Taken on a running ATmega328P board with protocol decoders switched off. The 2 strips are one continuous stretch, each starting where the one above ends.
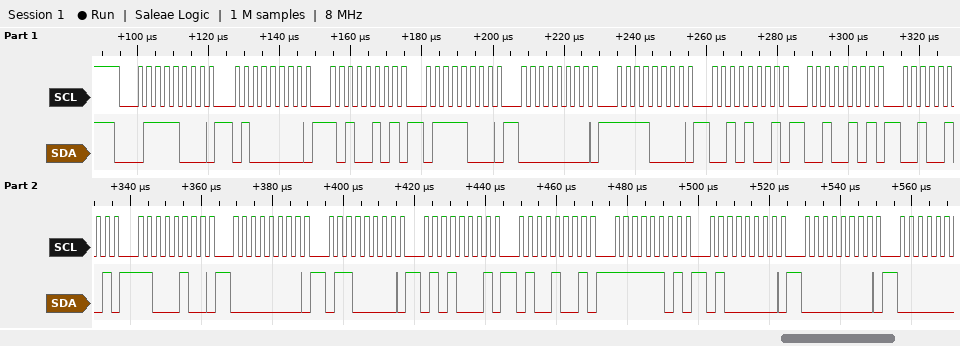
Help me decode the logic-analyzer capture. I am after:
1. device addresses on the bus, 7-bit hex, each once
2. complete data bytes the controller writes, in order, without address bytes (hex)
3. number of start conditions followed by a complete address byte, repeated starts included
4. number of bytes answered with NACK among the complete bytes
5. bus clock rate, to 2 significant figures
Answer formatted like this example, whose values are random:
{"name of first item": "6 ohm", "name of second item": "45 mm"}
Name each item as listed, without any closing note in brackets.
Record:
{"device addresses on the bus, 7-bit hex, each once": "0x3C", "complete data bytes the controller writes, in order, without address bytes": "40 A5 78 00 F0 29 25 25 C4 00 60 51 49 FD 40 00", "number of start conditions followed by a complete address byte, repeated starts included": "1", "number of bytes answered with NACK among the complete bytes": "0", "bus clock rate, to 2 significant figures": "400 kHz"}
